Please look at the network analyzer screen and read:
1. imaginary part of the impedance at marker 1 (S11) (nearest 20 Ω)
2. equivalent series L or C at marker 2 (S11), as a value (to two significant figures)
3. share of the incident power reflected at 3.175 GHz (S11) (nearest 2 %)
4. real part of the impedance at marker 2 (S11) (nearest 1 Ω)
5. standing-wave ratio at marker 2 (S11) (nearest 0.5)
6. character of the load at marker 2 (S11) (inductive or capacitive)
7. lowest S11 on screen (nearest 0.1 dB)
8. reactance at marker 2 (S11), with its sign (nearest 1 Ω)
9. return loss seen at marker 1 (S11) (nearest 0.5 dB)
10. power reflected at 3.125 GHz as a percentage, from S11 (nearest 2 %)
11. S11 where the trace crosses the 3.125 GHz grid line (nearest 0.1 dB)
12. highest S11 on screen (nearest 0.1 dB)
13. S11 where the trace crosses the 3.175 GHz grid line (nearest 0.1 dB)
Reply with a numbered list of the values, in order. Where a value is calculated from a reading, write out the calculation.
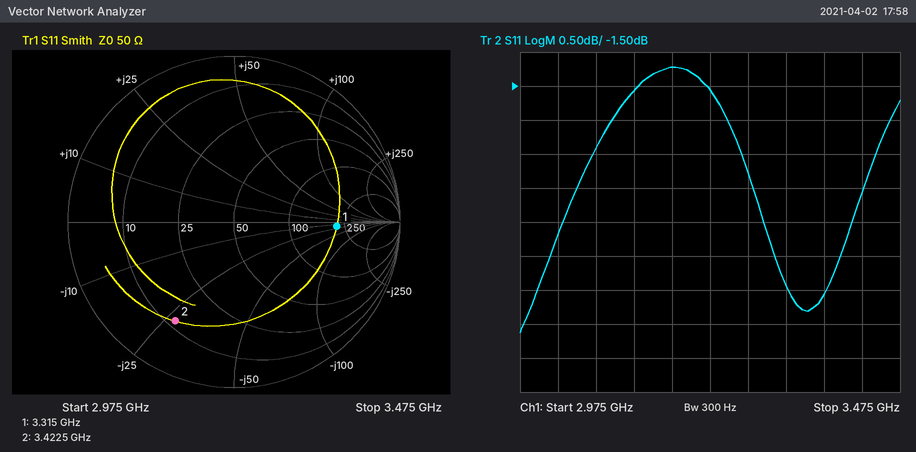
1. -20 Ω
2. C = 1/(2π × 3.4225 GHz × 27 Ω) ≈ 1.7 pF
3. 10^(-1.2/10) ≈ 76 %
4. 12 Ω
5. 5.5
6. capacitive
7. -5.1 dB
8. -27 Ω
9. 4.0 dB
10. 10^(-1.6/10) ≈ 69.2 %, so 70 % to the nearest 2 %
11. -1.6 dB
12. -1.2 dB
13. -1.2 dB
